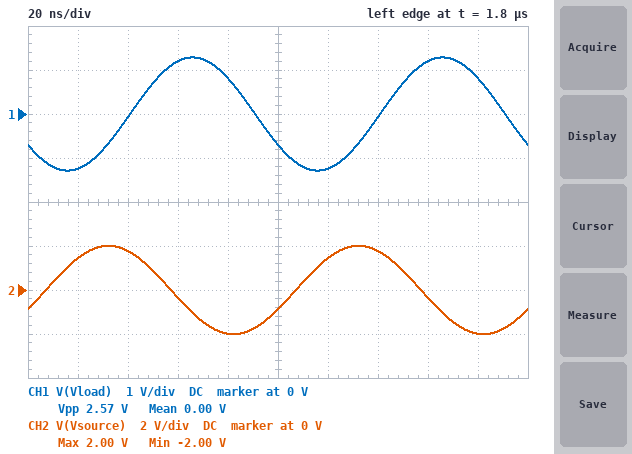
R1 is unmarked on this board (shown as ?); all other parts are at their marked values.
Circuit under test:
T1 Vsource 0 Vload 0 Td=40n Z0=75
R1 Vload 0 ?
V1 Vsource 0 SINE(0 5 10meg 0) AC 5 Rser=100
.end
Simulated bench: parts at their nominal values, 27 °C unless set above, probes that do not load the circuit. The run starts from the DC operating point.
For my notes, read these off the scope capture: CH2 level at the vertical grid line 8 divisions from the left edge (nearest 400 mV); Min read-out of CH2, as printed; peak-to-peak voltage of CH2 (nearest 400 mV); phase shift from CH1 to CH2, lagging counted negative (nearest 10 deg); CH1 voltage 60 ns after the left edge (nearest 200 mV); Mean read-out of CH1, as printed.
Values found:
-400 mV
-2.00 V
4.0 V
120 deg
1.2 V
0.00 V
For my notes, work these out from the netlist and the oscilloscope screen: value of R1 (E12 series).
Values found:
33 Ω
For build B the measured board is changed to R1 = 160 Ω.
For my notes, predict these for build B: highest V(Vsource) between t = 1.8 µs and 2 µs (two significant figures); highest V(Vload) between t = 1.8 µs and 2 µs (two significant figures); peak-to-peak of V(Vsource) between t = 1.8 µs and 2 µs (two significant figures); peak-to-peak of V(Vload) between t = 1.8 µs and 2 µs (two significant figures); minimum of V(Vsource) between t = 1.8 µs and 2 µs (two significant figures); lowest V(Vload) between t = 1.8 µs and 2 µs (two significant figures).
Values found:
2.5 V
3.0 V
5.1 V
5.9 V
-2.5 V
-3.0 V
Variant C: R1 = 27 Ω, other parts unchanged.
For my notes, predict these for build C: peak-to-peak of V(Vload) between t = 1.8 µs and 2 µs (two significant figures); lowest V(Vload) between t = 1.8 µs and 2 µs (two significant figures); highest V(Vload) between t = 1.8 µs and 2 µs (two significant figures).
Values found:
2.2 V
-1.1 V
1.1 V
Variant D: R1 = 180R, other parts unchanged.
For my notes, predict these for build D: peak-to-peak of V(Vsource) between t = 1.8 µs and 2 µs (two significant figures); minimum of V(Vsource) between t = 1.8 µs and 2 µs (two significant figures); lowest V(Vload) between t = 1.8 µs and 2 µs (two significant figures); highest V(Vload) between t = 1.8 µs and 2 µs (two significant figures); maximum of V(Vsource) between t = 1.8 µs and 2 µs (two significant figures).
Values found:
5.2 V
-2.6 V
-3.1 V
3.1 V
2.6 V
